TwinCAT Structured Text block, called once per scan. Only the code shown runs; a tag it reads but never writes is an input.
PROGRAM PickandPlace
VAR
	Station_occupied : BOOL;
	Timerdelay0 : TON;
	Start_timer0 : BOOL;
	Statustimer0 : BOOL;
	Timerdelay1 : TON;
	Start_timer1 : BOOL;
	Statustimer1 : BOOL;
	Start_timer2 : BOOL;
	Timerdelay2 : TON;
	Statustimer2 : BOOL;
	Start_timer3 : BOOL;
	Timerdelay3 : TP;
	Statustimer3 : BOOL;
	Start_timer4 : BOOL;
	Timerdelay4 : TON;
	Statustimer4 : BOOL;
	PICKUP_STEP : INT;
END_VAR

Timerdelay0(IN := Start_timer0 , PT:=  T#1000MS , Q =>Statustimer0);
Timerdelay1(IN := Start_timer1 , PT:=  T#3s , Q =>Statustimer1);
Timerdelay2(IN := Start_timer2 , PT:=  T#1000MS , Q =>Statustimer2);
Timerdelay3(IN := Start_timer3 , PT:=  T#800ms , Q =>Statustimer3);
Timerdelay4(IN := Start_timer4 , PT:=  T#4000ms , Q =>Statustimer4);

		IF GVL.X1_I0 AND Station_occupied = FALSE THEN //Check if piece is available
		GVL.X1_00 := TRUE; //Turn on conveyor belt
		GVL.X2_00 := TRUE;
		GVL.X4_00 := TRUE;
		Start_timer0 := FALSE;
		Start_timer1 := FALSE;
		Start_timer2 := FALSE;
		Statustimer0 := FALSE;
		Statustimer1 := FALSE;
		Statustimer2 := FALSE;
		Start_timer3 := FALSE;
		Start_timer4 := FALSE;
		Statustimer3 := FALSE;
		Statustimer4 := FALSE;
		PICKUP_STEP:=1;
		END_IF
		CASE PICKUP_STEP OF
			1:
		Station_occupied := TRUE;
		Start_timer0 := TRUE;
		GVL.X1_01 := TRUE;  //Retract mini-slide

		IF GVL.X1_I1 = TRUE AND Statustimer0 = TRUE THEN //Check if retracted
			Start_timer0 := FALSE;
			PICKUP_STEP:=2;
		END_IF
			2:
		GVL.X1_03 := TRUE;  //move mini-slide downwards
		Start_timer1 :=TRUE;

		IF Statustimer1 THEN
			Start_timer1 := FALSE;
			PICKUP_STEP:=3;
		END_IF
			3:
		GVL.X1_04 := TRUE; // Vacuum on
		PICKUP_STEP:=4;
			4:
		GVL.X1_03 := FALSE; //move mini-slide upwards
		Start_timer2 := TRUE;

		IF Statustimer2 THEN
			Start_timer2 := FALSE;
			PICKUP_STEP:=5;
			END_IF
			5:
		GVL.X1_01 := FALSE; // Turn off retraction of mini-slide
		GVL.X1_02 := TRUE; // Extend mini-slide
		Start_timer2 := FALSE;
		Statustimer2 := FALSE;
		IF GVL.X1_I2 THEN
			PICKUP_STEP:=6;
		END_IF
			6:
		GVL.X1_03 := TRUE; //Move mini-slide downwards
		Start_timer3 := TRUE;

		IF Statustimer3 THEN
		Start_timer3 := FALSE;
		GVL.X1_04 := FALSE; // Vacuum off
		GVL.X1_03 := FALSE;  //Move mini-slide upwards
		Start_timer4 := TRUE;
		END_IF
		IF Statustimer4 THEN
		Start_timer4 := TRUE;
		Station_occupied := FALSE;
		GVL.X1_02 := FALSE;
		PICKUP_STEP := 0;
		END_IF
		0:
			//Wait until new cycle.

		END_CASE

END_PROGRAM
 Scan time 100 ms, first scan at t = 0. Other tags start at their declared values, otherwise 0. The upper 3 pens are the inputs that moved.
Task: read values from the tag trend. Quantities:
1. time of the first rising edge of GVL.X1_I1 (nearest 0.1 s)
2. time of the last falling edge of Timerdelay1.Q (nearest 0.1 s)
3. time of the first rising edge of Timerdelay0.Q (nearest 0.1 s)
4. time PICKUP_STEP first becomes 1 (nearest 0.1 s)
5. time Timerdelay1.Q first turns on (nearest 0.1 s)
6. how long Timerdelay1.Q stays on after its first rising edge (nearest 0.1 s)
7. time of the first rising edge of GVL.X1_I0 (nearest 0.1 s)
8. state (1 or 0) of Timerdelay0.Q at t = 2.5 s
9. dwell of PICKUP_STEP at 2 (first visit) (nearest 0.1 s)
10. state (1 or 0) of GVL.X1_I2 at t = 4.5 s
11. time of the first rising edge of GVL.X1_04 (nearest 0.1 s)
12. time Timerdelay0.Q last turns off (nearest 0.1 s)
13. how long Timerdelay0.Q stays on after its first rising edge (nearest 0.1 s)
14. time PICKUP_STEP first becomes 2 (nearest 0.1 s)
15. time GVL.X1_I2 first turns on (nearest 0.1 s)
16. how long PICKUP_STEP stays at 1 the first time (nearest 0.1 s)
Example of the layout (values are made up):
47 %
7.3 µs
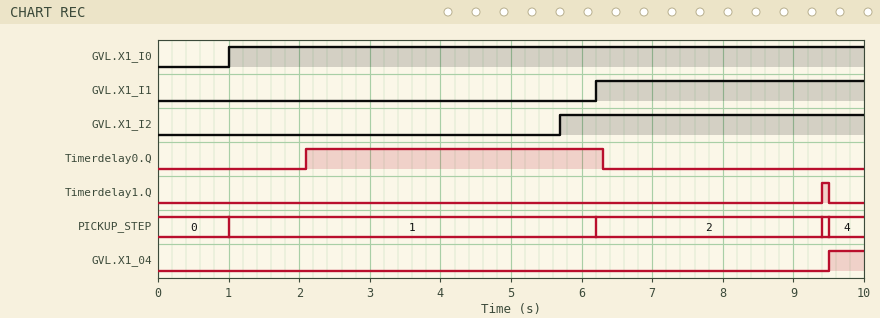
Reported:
6.2 s
9.5 s
2.1 s
1.0 s
9.4 s
0.1 s
1.0 s
1
3.2 s
0
9.5 s
6.3 s
4.2 s
6.2 s
5.7 s
5.2 s
